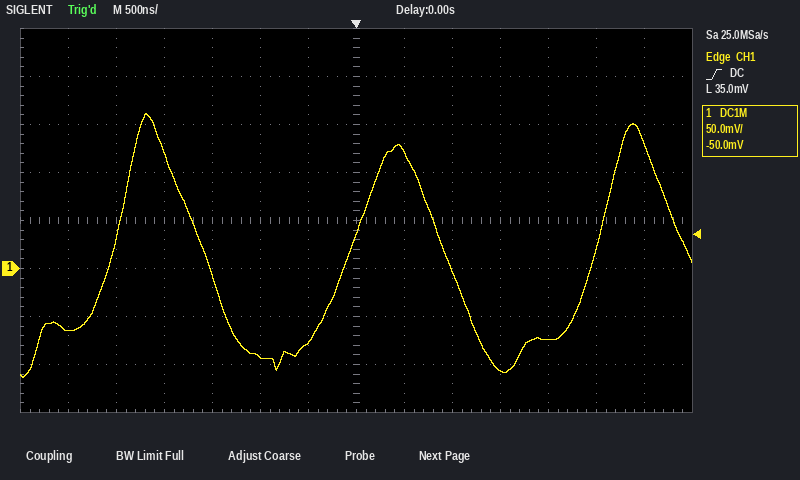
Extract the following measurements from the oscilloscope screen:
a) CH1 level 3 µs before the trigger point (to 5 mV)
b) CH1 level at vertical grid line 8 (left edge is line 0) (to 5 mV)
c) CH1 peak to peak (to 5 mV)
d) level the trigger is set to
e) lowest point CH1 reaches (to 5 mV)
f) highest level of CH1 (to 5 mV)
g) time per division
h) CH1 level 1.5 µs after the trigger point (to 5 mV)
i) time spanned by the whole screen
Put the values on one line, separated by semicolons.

-65 mV; 120 mV; 275 mV; 35.0 mV; -115 mV; 160 mV; 500 ns; -105 mV; 7 µs
